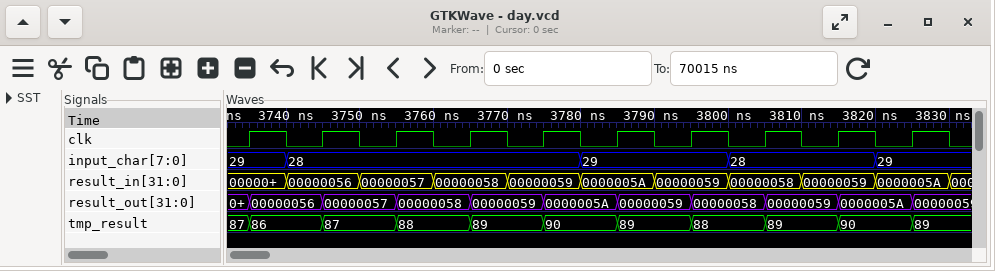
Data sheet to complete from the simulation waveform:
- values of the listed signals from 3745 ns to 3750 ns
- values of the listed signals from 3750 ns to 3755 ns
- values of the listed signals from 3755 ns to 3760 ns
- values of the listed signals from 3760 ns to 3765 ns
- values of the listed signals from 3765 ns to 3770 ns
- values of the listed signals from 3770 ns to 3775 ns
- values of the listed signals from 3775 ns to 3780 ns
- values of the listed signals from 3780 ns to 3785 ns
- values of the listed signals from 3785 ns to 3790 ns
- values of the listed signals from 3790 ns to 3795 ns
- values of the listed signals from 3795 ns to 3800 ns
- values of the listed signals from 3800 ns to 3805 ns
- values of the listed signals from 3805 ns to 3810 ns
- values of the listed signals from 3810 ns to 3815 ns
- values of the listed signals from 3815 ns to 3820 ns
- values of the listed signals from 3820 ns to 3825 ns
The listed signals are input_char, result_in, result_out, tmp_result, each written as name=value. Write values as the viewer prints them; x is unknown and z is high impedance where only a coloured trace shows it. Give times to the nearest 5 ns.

input_char=28, result_in=00000056, result_out=00000057, tmp_result=87
input_char=28, result_in=00000057, result_out=00000057, tmp_result=87
input_char=28, result_in=00000057, result_out=00000058, tmp_result=88
input_char=28, result_in=00000058, result_out=00000058, tmp_result=88
input_char=28, result_in=00000058, result_out=00000059, tmp_result=89
input_char=28, result_in=00000059, result_out=00000059, tmp_result=89
input_char=28, result_in=00000059, result_out=0000005A, tmp_result=90
input_char=29, result_in=0000005A, result_out=0000005A, tmp_result=90
input_char=29, result_in=0000005A, result_out=00000059, tmp_result=89
input_char=29, result_in=00000059, result_out=00000059, tmp_result=89
input_char=29, result_in=00000059, result_out=00000058, tmp_result=88
input_char=28, result_in=00000058, result_out=00000058, tmp_result=88
input_char=28, result_in=00000058, result_out=00000059, tmp_result=89
input_char=28, result_in=00000059, result_out=00000059, tmp_result=89
input_char=28, result_in=00000059, result_out=0000005A, tmp_result=90
input_char=29, result_in=0000005A, result_out=0000005A, tmp_result=90
